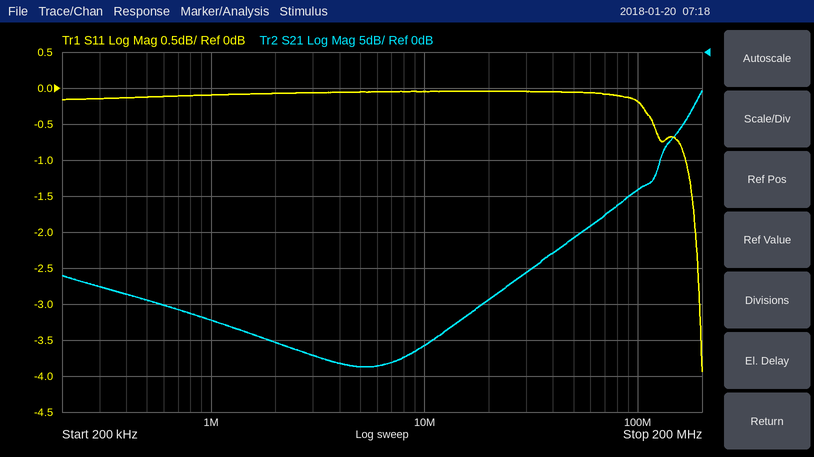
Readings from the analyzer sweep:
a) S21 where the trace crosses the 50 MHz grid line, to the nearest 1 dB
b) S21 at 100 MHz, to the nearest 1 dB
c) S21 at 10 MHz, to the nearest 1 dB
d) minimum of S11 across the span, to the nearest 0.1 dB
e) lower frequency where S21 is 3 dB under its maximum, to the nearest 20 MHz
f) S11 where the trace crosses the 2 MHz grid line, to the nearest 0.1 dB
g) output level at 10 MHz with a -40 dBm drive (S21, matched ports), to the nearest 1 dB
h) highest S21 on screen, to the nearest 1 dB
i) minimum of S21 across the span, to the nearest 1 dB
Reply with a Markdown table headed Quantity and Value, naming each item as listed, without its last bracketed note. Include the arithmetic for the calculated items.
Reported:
| Quantity | Value |
|---|---|
| S21 where the trace crosses the 50 MHz grid line, to the nearest 1 dB | -26 dB |
| S21 at 100 MHz, to the nearest 1 dB | -19 dB |
| S21 at 10 MHz, to the nearest 1 dB | -41 dB |
| minimum of S11 across the span, to the nearest 0.1 dB | -3.9 dB |
| lower frequency where S21 is 3 dB under its maximum, to the nearest 20 MHz | 180 MHz |
| S11 where the trace crosses the 2 MHz grid line, to the nearest 0.1 dB | -0.1 dB |
| output level at 10 MHz with a -40 dBm drive (S21, matched ports), to the nearest 1 dB | -40 dBm + (-41 dB) = -81 dBm |
| highest S21 on screen, to the nearest 1 dB | -5 dB |
| minimum of S21 across the span, to the nearest 1 dB | -44 dB |
